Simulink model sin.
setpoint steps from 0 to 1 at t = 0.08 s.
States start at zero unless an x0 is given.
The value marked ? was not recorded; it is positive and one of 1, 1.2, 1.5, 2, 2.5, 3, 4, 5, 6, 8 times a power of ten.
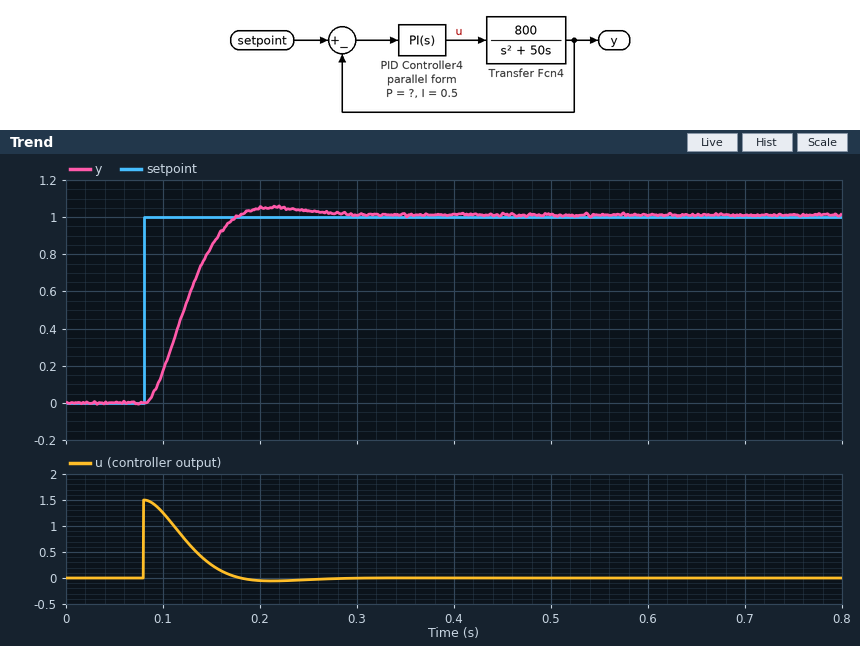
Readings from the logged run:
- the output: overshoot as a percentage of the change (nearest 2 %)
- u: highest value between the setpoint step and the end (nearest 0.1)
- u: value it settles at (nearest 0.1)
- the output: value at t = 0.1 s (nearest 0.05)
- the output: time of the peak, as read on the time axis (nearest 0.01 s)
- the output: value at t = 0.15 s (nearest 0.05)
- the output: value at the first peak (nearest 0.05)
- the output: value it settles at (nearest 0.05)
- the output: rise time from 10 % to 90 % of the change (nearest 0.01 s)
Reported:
4 %
1.5
0.0
0.15
0.21 s
0.85
1.05
1.00
0.06 s
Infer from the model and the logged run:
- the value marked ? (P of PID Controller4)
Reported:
1.5
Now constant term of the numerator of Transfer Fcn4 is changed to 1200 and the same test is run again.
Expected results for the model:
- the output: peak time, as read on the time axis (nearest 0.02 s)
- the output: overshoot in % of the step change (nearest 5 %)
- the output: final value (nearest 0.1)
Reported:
0.18 s
10 %
1.0
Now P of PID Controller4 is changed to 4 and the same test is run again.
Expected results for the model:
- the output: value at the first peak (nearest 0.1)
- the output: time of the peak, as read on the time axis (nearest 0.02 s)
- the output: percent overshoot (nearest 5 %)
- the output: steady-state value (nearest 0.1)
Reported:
1.2
0.14 s
20 %
1.0
